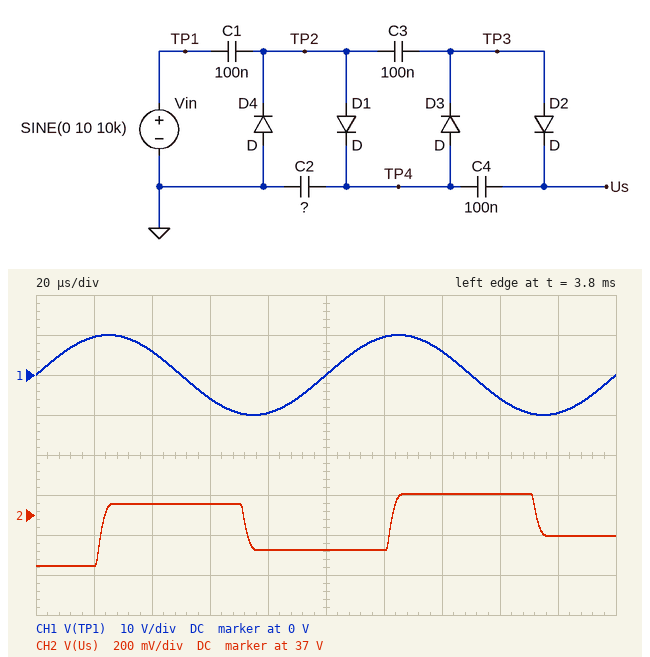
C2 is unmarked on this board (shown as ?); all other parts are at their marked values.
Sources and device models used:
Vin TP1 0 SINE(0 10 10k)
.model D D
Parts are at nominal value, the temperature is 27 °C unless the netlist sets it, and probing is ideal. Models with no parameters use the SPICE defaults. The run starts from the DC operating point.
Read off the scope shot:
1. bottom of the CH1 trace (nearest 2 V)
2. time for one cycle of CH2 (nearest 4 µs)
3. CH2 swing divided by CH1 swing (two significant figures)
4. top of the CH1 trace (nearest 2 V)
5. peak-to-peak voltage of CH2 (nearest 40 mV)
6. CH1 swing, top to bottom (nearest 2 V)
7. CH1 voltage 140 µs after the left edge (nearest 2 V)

-10 V
100 µs
0.018
10 V
360 mV
20 V
6 V
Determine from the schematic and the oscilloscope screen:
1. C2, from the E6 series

33 nF
